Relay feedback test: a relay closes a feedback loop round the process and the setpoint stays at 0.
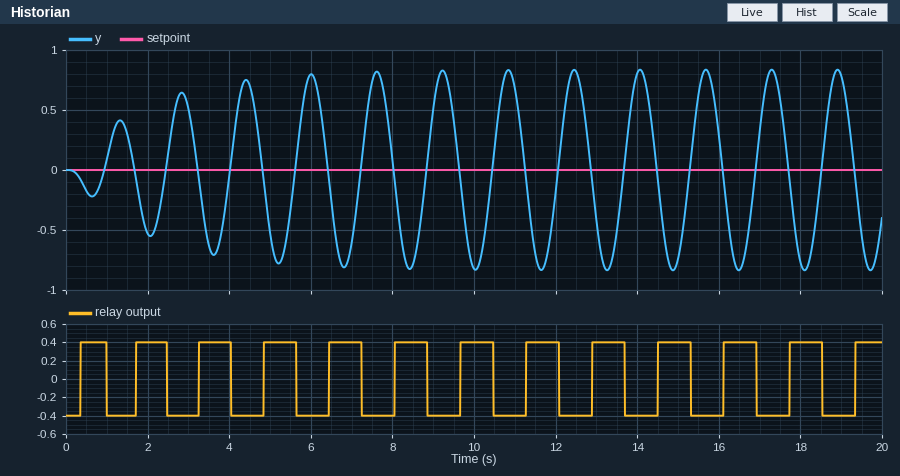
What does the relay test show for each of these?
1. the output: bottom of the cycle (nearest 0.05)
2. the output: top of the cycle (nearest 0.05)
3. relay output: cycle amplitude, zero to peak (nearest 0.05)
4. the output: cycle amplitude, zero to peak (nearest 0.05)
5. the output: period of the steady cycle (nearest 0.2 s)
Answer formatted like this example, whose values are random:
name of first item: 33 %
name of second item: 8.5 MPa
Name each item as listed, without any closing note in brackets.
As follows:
the output: bottom of the cycle: -0.85
the output: top of the cycle: 0.85
relay output: cycle amplitude, zero to peak: 0.40
the output: cycle amplitude, zero to peak: 0.85
the output: period of the steady cycle: 1.6 s
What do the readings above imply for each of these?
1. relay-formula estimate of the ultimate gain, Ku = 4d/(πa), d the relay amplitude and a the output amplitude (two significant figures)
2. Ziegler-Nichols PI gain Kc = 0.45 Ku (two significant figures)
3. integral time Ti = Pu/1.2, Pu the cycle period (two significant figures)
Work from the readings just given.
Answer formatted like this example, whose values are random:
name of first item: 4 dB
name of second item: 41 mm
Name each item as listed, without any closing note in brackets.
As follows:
relay-formula estimate of the ultimate gain, Ku = 4d/(πa), d the relay amplitude and a the output amplitude: 0.60
Ziegler-Nichols PI gain Kc = 0.45 Ku: 0.27
integral time Ti = Pu/1.2, Pu the cycle period: 1.3 s
